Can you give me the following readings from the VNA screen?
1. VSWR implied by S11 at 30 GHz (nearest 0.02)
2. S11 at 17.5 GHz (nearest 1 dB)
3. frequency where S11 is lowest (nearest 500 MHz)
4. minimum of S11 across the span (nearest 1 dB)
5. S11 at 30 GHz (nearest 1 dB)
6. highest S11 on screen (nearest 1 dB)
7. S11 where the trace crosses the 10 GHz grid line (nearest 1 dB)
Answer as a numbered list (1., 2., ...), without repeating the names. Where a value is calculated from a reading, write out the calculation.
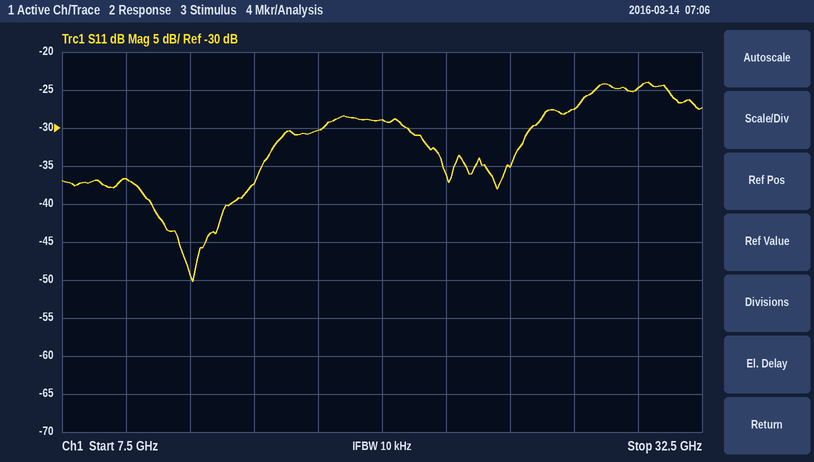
1. |Γ| = 10^(-25/20) = 0.0562; VSWR = (1 + 0.0562)/(1 − 0.0562) ≈ 1.12
2. -30 dB
3. 12.5 GHz
4. -50 dB
5. -25 dB
6. -24 dB
7. -37 dB
